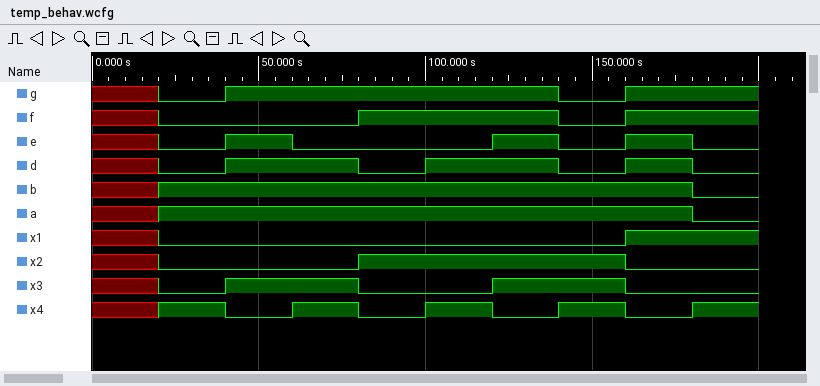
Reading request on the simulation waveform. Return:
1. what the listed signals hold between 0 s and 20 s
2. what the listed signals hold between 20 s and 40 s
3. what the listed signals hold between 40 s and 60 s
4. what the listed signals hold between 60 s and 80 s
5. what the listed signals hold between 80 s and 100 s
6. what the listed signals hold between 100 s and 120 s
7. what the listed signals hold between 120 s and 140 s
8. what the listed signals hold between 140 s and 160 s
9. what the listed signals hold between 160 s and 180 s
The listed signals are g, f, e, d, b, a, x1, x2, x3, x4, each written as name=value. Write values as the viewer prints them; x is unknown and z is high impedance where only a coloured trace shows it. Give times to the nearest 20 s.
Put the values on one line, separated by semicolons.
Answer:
g=x, f=x, e=x, d=x, b=x, a=x, x1=x, x2=x, x3=x, x4=x; g=0, f=0, e=0, d=0, b=1, a=1, x1=0, x2=0, x3=0, x4=1; g=1, f=0, e=1, d=1, b=1, a=1, x1=0, x2=0, x3=1, x4=0; g=1, f=0, e=0, d=1, b=1, a=1, x1=0, x2=0, x3=1, x4=1; g=1, f=1, e=0, d=0, b=1, a=1, x1=0, x2=1, x3=0, x4=0; g=1, f=1, e=0, d=1, b=1, a=1, x1=0, x2=1, x3=0, x4=1; g=1, f=1, e=1, d=1, b=1, a=1, x1=0, x2=1, x3=1, x4=0; g=0, f=0, e=0, d=0, b=1, a=1, x1=0, x2=1, x3=1, x4=1; g=1, f=1, e=1, d=1, b=1, a=1, x1=1, x2=0, x3=0, x4=0
